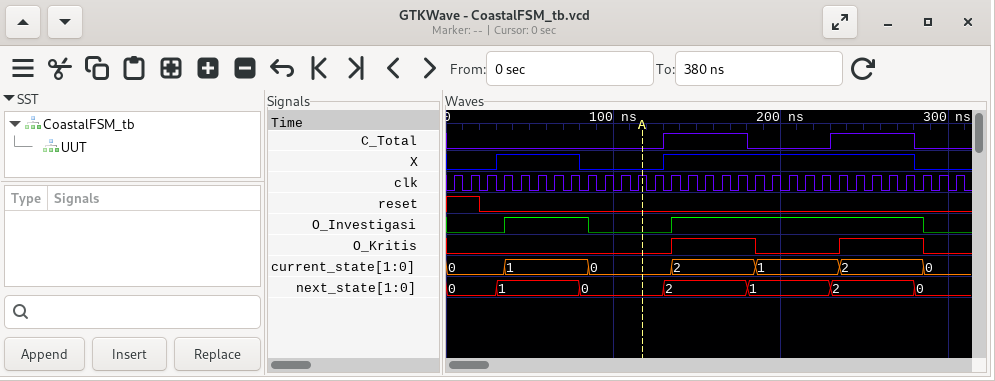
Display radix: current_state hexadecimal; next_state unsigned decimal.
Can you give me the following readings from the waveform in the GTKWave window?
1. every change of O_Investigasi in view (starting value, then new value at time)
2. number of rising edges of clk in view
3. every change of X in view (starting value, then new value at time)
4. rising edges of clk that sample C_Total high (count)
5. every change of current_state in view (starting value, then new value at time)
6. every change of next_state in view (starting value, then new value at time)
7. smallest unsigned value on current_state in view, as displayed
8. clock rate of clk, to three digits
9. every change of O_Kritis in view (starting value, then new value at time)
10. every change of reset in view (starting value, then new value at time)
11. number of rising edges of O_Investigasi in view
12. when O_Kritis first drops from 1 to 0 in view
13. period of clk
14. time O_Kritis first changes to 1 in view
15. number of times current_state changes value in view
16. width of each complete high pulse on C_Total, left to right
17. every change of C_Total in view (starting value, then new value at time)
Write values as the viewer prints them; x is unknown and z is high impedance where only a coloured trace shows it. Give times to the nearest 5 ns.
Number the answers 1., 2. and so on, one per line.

1. 0, 1 at 35 ns, 0 at 85 ns, 1 at 135 ns, 0 at 285 ns
2. 31
3. 0, 1 at 30 ns, 0 at 80 ns, 1 at 130 ns, 0 at 280 ns
4. 10
5. 0, 1 at 35 ns, 0 at 85 ns, 2 at 135 ns, 1 at 185 ns, 2 at 235 ns, 0 at 285 ns
6. 0, 1 at 30 ns, 0 at 80 ns, 2 at 130 ns, 1 at 180 ns, 2 at 230 ns, 0 at 280 ns
7. 0
8. 100 MHz
9. 0, 1 at 135 ns, 0 at 185 ns, 1 at 235 ns, 0 at 285 ns
10. 1, 0 at 20 ns
11. 2
12. 185 ns
13. 10 ns
14. 135 ns
15. 6
16. 50 ns, 50 ns
17. 0, 1 at 130 ns, 0 at 180 ns, 1 at 230 ns, 0 at 280 ns
